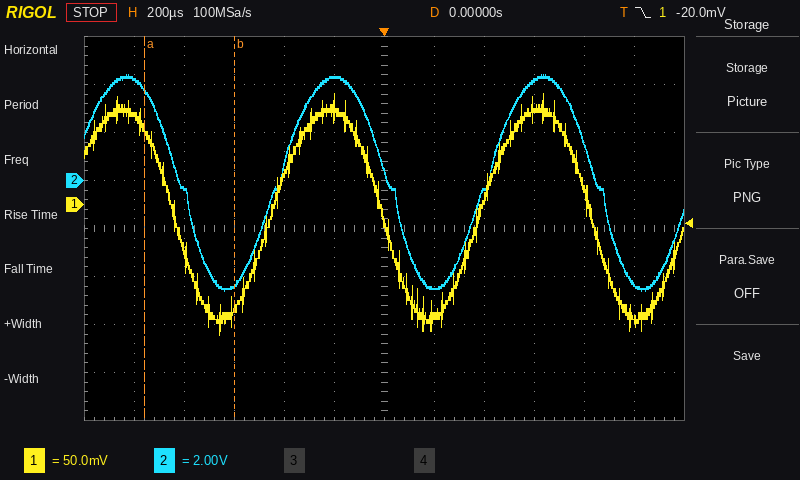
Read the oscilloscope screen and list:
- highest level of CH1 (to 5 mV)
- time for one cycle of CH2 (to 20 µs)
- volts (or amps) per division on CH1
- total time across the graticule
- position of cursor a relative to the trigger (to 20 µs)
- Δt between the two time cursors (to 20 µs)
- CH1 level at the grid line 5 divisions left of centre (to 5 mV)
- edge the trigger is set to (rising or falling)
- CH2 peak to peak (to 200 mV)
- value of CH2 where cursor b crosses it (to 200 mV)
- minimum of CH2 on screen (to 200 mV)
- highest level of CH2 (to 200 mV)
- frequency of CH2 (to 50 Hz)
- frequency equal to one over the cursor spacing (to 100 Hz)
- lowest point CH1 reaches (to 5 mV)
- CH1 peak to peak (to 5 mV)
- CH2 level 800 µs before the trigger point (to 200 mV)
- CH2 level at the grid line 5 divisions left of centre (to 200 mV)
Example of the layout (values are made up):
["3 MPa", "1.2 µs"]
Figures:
["115 mV", "840 µs", "50 mV", "2.4 ms", "-960 µs", "360 µs", "90 mV", "falling", "9.0 V", "-4.4 V", "-4.6 V", "4.4 V", "1.20 kHz", "2.8 kHz", "-135 mV", "250 mV", "-400 mV", "4.2 V"]
